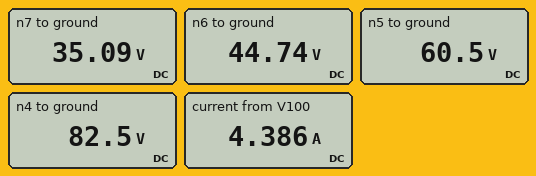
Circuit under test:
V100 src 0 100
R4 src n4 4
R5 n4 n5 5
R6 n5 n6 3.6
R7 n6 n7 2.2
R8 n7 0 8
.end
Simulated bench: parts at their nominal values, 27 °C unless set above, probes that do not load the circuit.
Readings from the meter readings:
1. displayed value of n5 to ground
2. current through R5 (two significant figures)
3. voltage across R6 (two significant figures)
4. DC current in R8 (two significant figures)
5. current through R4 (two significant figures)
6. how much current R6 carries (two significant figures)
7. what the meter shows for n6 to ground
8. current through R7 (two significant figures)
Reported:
60.5 V
4.4 A
16 V
4.4 A
4.4 A
4.4 A
44.74 V
4.4 A
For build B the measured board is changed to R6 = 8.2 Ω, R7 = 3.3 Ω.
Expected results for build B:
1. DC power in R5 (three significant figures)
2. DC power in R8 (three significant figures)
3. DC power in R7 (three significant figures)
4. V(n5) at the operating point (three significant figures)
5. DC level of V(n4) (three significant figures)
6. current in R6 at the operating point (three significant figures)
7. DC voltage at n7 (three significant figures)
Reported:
61.6 W
98.5 W
40.6 W
68.4 V
86.0 V
3.51 A
28.1 V
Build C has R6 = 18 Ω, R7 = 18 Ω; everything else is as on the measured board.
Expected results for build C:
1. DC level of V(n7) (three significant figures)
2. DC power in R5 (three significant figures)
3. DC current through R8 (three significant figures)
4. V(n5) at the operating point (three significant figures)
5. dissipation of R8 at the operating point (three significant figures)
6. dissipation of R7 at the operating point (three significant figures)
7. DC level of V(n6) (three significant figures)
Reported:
15.1 V
17.8 W
1.89 A
83.0 V
28.5 W
64.1 W
49.1 V
